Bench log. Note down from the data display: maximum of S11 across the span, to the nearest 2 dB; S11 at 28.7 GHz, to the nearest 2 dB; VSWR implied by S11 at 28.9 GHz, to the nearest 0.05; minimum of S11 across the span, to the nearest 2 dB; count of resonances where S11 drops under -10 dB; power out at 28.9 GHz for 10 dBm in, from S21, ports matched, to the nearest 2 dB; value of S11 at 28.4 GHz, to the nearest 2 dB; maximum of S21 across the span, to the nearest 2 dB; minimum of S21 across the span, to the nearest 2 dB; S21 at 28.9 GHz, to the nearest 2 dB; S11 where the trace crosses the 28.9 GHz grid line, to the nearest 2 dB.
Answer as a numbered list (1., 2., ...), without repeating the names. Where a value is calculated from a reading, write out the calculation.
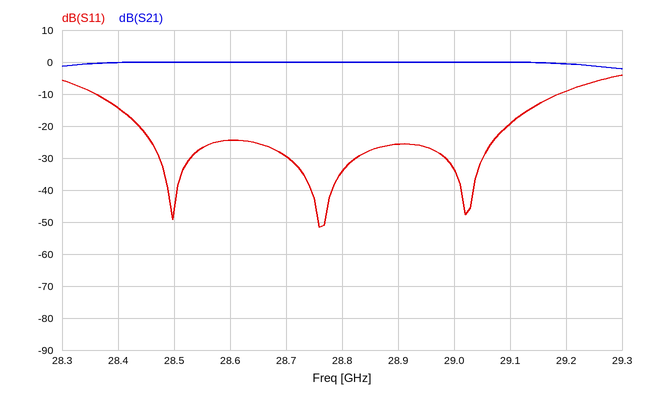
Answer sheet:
1. -4 dB
2. -30 dB
3. |Γ| = 10^(-26/20) = 0.0501; VSWR = (1 + 0.0501)/(1 − 0.0501) ≈ 1.11, so 1.10 to the nearest 0.05
4. -52 dB
5. 3
6. 10 dBm + (0 dB) = 10 dBm
7. -14 dB
8. 0 dB
9. -2 dB
10. 0 dB
11. -26 dB
